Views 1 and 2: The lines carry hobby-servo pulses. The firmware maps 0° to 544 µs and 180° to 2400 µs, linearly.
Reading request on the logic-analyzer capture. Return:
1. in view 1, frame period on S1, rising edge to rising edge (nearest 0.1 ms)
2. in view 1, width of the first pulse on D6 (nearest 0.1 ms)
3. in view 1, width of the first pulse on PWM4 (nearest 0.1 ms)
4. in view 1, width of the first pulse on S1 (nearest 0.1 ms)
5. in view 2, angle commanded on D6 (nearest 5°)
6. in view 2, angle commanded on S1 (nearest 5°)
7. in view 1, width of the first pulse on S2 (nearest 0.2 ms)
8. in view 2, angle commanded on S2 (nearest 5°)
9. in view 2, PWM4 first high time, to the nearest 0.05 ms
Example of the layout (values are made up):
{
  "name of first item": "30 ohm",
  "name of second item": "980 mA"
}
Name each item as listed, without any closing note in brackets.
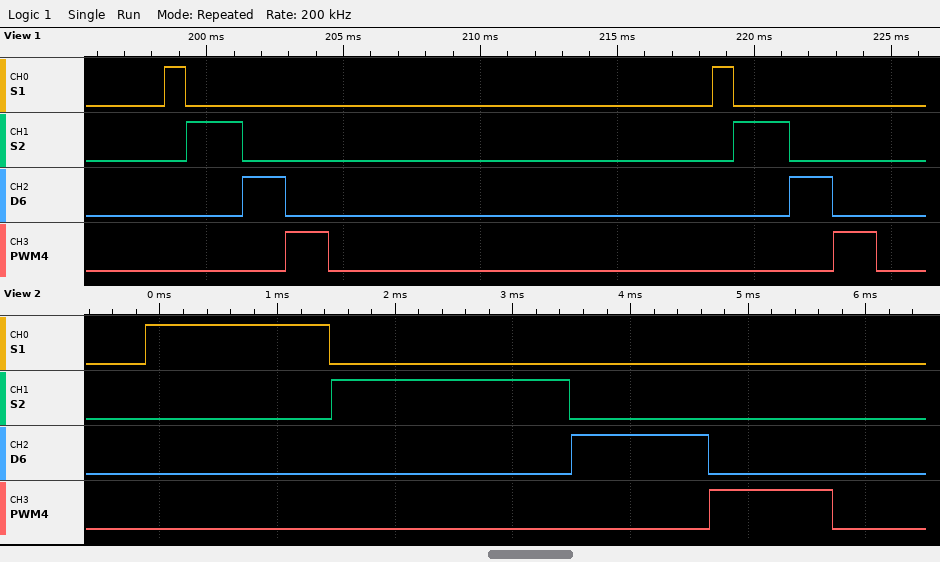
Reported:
{
  "in view 1, frame period on S1, rising edge to rising edge": "20.0 ms",
  "in view 1, width of the first pulse on D6": "1.6 ms",
  "in view 1, width of the first pulse on PWM4": "1.6 ms",
  "in view 1, width of the first pulse on S1": "0.8 ms",
  "in view 2, angle commanded on D6": "60°",
  "in view 2, angle commanded on S1": "100°",
  "in view 1, width of the first pulse on S2": "2.0 ms",
  "in view 2, angle commanded on S2": "145°",
  "in view 2, PWM4 first high time, to the nearest 0.05 ms": "1.05 ms"
}
